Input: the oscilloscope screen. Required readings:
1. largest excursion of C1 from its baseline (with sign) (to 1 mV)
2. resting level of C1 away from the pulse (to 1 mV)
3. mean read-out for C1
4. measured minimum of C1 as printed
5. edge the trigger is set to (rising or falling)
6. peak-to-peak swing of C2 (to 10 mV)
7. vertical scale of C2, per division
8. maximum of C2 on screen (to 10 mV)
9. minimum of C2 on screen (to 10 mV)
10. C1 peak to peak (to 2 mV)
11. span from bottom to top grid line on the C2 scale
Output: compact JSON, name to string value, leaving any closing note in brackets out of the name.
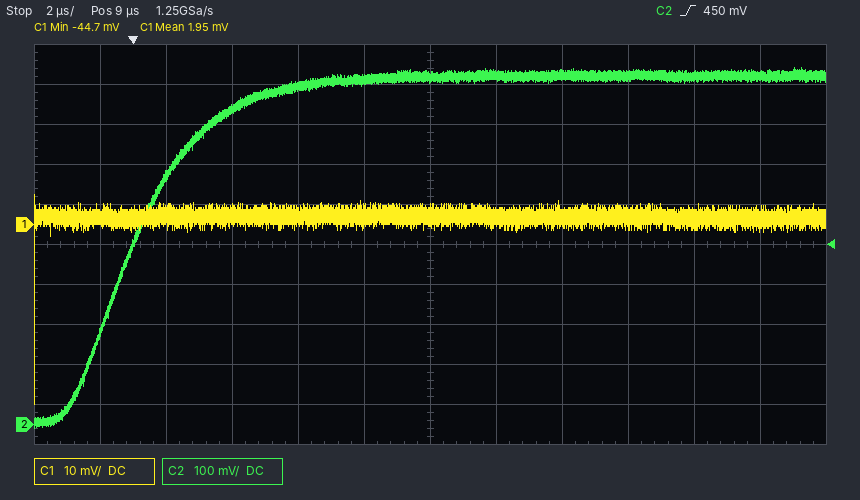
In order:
{"largest excursion of C1 from its baseline (with sign)": "-47 mV", "resting level of C1 away from the pulse": "2 mV", "mean read-out for C1": "1.95 mV", "measured minimum of C1 as printed": "-44.7 mV", "edge the trigger is set to": "rising", "peak-to-peak swing of C2": "900 mV", "vertical scale of C2, per division": "100 mV", "maximum of C2 on screen": "890 mV", "minimum of C2 on screen": "-10 mV", "C1 peak to peak": "52 mV", "span from bottom to top grid line on the C2 scale": "1 V"}
